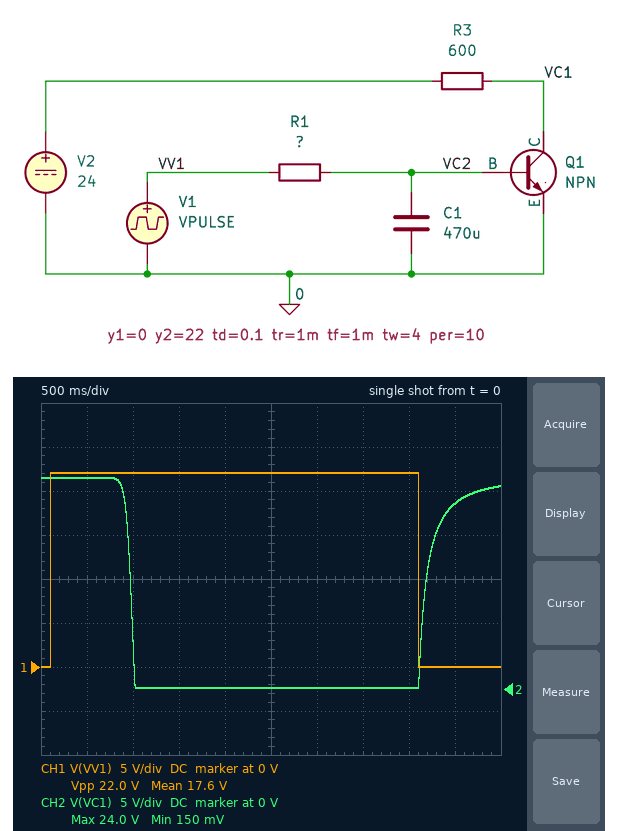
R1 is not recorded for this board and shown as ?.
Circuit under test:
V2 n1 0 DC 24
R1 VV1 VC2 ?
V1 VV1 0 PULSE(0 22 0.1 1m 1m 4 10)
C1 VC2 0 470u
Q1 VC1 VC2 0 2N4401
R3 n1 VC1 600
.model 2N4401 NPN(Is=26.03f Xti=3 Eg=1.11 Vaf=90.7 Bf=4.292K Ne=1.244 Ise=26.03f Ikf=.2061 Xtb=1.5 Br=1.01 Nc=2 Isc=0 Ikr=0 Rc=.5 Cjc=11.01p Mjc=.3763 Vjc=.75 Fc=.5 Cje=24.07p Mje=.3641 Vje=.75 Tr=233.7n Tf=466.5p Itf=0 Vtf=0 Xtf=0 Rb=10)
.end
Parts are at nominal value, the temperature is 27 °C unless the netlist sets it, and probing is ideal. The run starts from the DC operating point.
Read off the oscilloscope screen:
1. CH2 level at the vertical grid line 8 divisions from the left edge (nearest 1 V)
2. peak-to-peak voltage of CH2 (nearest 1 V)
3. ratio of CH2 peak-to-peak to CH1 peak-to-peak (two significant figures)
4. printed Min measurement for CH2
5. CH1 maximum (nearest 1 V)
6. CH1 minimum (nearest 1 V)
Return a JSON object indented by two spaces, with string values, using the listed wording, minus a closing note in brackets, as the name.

{
  "CH2 level at the vertical grid line 8 divisions from the left edge": "0 V",
  "peak-to-peak voltage of CH2": "24 V",
  "ratio of CH2 peak-to-peak to CH1 peak-to-peak": "1.1",
  "printed Min measurement for CH2": "150 mV",
  "CH1 maximum": "22 V",
  "CH1 minimum": "0 V"
}
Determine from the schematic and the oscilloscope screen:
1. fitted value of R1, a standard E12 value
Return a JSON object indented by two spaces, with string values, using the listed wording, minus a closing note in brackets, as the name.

{
  "fitted value of R1, a standard E12 value": "56 kΩ"
}
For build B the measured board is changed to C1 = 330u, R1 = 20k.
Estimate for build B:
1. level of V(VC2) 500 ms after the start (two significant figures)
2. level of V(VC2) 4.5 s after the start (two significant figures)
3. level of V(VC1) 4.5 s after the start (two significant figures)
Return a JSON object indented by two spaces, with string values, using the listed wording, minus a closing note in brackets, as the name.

{
  "level of V(VC2) 500 ms after the start": "740 mV",
  "level of V(VC2) 4.5 s after the start": "640 mV",
  "level of V(VC1) 4.5 s after the start": "23 V"
}
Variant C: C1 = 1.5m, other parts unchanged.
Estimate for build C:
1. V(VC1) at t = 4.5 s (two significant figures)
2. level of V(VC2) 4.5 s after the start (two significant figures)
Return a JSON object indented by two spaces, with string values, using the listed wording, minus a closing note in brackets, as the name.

{
  "V(VC1) at t = 4.5 s": "15 V",
  "level of V(VC2) 4.5 s after the start": "700 mV"
}
